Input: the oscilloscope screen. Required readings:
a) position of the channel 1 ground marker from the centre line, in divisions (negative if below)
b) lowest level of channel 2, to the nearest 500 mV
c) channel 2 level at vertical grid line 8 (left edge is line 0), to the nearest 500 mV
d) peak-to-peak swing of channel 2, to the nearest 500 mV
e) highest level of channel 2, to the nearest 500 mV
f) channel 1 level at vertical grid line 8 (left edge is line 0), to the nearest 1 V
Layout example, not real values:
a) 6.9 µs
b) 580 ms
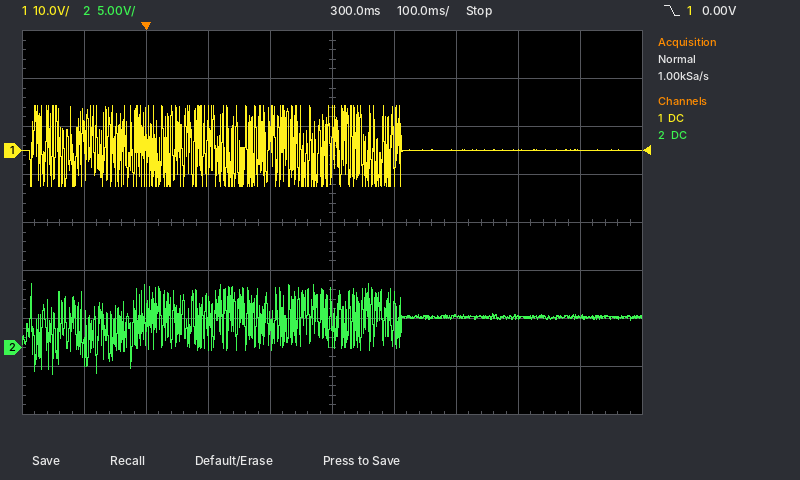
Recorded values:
a) +1.5 div
b) -3.0 V
c) 3.0 V
d) 9.5 V
e) 6.5 V
f) 0 V
